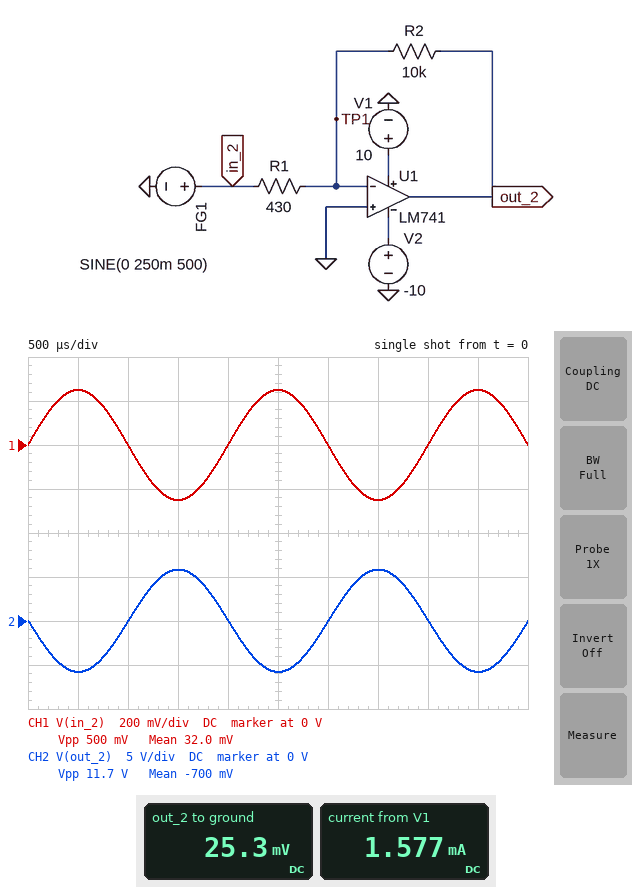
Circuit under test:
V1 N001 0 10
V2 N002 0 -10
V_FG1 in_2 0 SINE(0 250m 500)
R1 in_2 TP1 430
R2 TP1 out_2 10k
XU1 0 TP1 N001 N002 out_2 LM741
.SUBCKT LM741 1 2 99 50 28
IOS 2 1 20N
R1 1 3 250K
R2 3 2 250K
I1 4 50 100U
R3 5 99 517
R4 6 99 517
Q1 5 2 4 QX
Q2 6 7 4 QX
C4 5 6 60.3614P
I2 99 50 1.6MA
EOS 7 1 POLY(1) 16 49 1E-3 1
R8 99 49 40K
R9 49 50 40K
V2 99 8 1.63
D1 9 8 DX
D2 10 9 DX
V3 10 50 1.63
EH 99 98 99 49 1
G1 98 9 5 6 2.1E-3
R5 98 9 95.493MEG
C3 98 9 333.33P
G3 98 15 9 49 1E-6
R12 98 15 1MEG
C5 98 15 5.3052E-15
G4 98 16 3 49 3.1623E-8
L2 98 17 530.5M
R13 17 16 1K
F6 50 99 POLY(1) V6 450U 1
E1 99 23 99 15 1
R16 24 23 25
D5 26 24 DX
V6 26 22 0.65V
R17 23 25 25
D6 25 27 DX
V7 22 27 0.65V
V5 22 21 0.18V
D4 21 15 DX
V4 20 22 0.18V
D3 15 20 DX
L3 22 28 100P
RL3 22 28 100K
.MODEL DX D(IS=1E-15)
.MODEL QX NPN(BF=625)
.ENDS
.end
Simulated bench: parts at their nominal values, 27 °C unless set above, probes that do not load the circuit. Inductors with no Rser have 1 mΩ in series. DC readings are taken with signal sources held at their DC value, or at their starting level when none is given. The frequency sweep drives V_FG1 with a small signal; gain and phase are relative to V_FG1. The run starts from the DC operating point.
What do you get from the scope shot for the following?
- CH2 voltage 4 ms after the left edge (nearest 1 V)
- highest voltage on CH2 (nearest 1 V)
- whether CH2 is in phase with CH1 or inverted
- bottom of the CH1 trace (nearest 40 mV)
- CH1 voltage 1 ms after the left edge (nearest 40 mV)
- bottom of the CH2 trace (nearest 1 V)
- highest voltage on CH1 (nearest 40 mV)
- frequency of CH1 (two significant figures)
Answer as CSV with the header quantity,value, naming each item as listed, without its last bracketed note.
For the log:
quantity,value
CH2 voltage 4 ms after the left edge,0 V
highest voltage on CH2,6 V
whether CH2 is in phase with CH1 or inverted,inverted
bottom of the CH1 trace,-240 mV
CH1 voltage 1 ms after the left edge,0 V
bottom of the CH2 trace,-6 V
highest voltage on CH1,240 mV
frequency of CH1,500 Hz
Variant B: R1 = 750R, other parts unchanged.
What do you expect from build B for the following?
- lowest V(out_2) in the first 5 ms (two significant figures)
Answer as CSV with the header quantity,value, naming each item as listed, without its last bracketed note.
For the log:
quantity,value
lowest V(out_2) in the first 5 ms,-3.3 V
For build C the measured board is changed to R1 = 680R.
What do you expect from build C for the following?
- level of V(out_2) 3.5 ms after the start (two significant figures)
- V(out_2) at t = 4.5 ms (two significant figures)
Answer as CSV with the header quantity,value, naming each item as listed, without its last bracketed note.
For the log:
quantity,value
level of V(out_2) 3.5 ms after the start,3.7 V
V(out_2) at t = 4.5 ms,-3.7 V
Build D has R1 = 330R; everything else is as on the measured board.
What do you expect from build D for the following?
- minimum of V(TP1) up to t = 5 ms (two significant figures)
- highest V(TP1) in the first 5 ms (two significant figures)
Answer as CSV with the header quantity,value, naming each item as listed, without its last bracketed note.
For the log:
quantity,value
minimum of V(TP1) up to t = 5 ms,-2.9 mV
highest V(TP1) in the first 5 ms,4.9 mV
